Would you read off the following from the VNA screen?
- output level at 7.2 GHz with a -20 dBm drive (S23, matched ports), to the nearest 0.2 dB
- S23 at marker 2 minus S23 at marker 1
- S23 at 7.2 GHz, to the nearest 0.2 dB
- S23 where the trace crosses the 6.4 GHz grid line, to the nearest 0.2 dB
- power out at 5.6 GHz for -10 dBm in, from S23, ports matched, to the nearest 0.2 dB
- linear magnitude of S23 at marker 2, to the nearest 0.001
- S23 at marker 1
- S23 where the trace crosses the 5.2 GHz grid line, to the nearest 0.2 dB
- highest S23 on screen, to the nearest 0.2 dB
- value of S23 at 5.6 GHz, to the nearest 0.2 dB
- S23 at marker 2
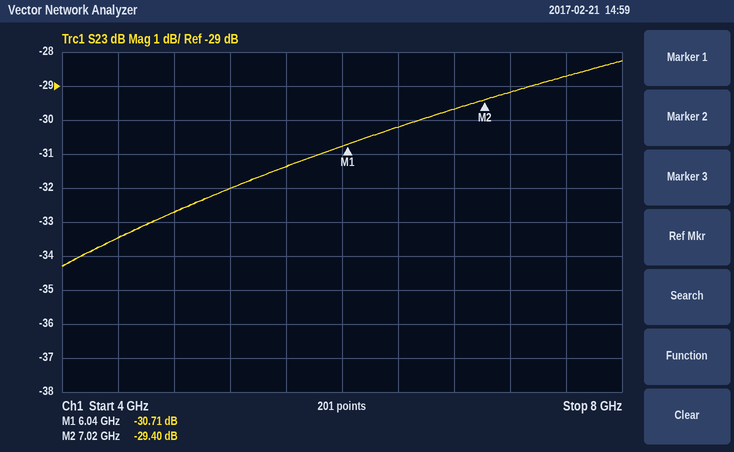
-49.2 dBm
1.31 dB
-29.2 dB
-30.2 dB
-41.4 dBm
0.034
-30.71 dB
-32.0 dB
-28.2 dB
-31.4 dB
-29.40 dB
